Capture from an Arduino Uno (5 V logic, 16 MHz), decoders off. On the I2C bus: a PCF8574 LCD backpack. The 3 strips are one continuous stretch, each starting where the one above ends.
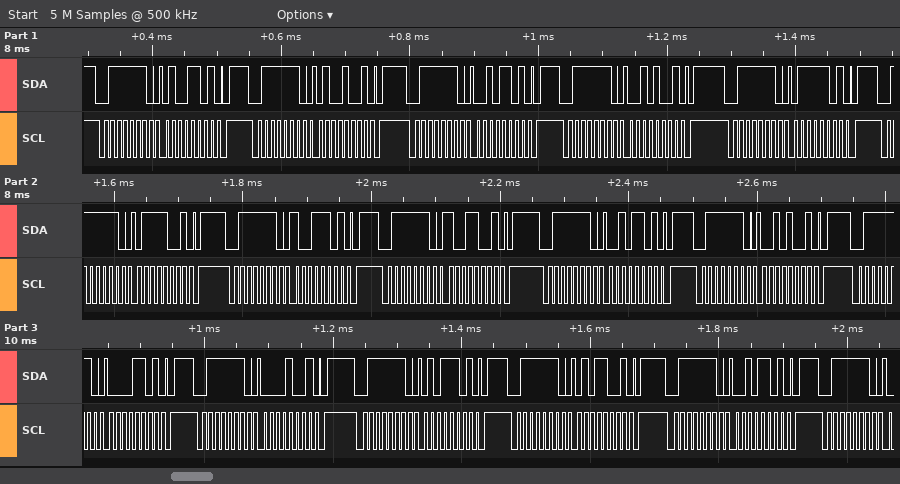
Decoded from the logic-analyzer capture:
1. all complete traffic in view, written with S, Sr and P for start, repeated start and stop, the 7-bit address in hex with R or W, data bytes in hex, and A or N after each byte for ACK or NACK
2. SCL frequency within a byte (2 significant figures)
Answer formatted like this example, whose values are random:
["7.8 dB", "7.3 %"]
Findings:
["S 3FW A 4D A P S 3FW A 49 A P S 3FW A 2D A P S 3FW A 29 A P S 3FW A 7D A P S 3FW A 79 A P S 3FW A 9D A P S 3FW A 99 A P S 3FW A 2D A P S 3FW A 29 A P S 3FW A 0D A P S 3FW A 09 A P S 3FW A 5D A P S 3FW A 59 A P S 3FW A 2D A P S 3FW A", "100 kHz"]
